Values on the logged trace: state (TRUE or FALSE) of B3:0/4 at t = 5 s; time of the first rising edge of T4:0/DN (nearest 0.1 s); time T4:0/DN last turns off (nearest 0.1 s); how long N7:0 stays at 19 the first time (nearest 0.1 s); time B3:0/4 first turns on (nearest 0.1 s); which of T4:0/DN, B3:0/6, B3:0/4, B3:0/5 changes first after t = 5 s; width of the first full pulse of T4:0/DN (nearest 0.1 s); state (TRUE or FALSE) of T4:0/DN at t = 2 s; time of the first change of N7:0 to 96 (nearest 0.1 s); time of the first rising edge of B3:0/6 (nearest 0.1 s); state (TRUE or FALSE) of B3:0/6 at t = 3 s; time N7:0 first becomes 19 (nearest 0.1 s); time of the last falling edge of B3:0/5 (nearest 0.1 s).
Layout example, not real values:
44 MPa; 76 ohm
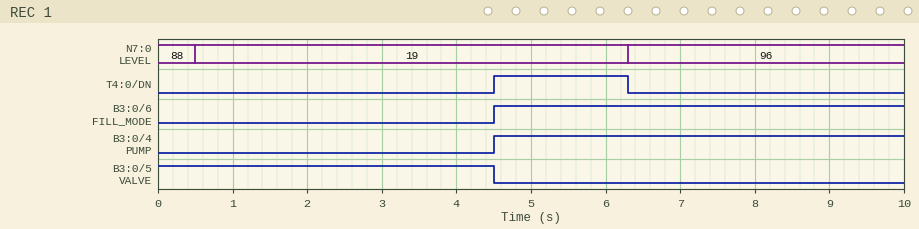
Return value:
TRUE; 4.5 s; 6.3 s; 5.8 s; 4.5 s; T4:0/DN; 1.8 s; FALSE; 6.3 s; 4.5 s; FALSE; 0.5 s; 4.5 s
